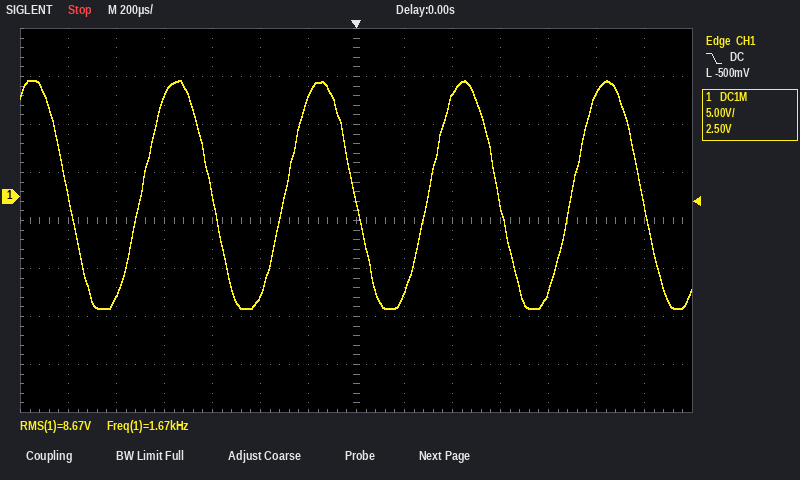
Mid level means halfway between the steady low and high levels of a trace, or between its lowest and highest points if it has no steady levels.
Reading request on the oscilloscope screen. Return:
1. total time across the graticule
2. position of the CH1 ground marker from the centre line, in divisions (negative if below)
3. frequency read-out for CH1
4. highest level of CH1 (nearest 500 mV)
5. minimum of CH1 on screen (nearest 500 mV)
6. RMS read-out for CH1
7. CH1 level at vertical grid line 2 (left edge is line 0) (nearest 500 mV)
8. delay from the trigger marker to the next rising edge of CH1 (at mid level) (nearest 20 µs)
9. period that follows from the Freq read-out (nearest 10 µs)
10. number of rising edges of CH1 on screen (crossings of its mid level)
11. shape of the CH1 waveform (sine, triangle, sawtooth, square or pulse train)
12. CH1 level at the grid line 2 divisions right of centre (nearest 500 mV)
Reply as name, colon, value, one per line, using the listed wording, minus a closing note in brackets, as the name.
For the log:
total time across the graticule: 2.8 ms
position of the CH1 ground marker from the centre line, in divisions: +0.5 div
frequency read-out for CH1: 1.67 kHz
highest level of CH1: 12.0 V
minimum of CH1 on screen: -11.5 V
RMS read-out for CH1: 8.67 V
CH1 level at vertical grid line 2 (left edge is line 0): -10.5 V
delay from the trigger marker to the next rising edge of CH1 (at mid level): 300 µs
period that follows from the Freq read-out: 600 µs
number of rising edges of CH1 on screen: 4
shape of the CH1 waveform: sine
CH1 level at the grid line 2 divisions right of centre: 10.5 V
